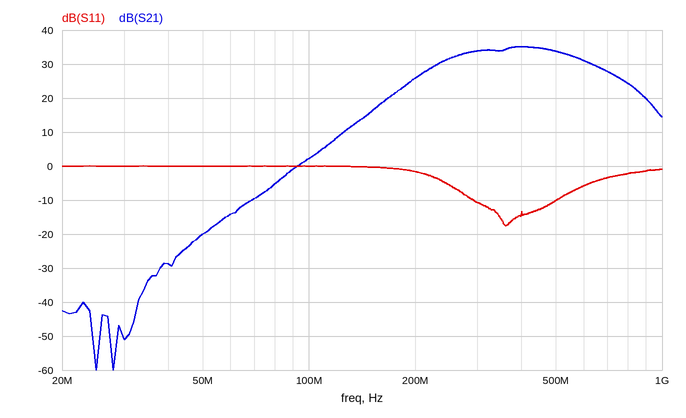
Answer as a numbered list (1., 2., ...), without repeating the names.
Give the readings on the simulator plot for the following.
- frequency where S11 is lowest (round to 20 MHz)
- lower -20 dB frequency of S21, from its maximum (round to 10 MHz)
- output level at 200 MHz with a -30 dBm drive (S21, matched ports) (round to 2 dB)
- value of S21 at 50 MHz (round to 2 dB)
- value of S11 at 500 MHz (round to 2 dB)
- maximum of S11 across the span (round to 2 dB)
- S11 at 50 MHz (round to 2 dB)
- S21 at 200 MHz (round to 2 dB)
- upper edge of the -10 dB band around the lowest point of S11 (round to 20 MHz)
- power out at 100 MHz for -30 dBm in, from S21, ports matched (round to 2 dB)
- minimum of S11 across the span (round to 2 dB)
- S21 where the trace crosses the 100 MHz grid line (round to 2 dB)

1. 360 MHz
2. 150 MHz
3. -4 dBm
4. -20 dB
5. -10 dB
6. 0 dB
7. 0 dB
8. 26 dB
9. 500 MHz
10. -28 dBm
11. -18 dB
12. 2 dB
